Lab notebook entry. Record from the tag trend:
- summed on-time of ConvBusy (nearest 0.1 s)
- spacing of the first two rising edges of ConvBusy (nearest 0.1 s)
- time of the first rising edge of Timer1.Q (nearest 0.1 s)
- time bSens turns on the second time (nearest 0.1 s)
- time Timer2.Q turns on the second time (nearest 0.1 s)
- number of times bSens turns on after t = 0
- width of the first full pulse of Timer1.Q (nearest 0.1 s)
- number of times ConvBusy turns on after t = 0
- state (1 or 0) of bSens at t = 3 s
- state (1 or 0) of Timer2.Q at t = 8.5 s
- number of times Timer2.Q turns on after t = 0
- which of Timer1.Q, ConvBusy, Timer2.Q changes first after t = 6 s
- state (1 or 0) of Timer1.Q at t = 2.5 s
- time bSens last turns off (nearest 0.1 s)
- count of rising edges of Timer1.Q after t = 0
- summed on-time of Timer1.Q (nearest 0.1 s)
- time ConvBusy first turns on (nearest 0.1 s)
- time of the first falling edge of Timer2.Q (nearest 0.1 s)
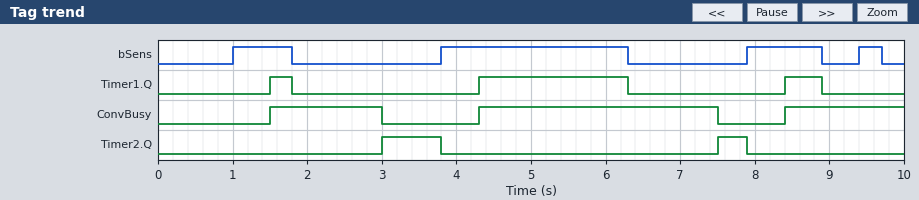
6.3 s
2.8 s
1.5 s
3.8 s
7.5 s
4
0.3 s
3
0
0
2
Timer1.Q
0
9.7 s
3
2.8 s
1.5 s
3.8 s
